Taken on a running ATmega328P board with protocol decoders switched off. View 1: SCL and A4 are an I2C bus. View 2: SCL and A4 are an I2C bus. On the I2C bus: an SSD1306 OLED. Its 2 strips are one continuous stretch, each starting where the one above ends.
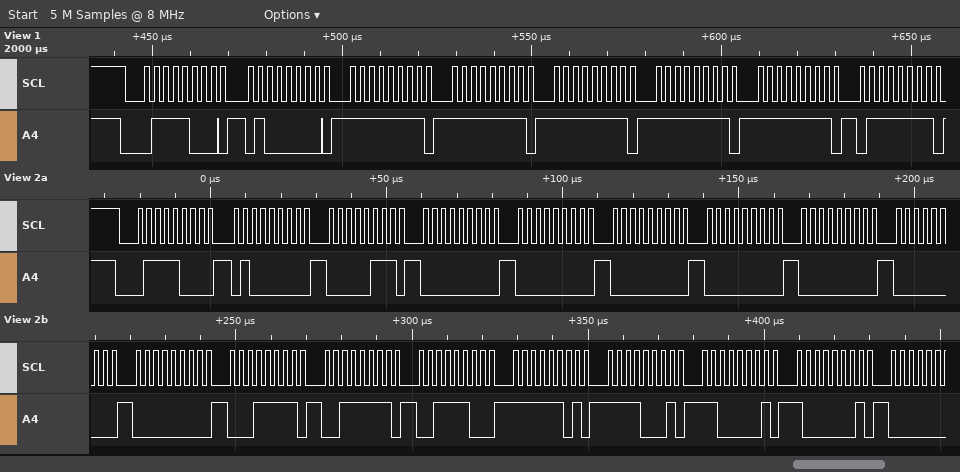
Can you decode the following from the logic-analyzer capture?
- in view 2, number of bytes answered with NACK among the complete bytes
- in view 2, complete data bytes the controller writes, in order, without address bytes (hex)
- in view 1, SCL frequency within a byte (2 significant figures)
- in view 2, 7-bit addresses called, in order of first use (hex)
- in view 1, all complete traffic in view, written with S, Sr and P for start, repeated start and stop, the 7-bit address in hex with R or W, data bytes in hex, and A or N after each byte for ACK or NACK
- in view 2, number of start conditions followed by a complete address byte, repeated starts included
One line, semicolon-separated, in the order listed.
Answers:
0; 40 07 00 00 00 00 00 00 00 1F 3F 3C FD F1 C1 81; 400 kHz; 0x3C; S 3CW A 40 A FF A FF A FF A FF A FF A 7F A; 1
